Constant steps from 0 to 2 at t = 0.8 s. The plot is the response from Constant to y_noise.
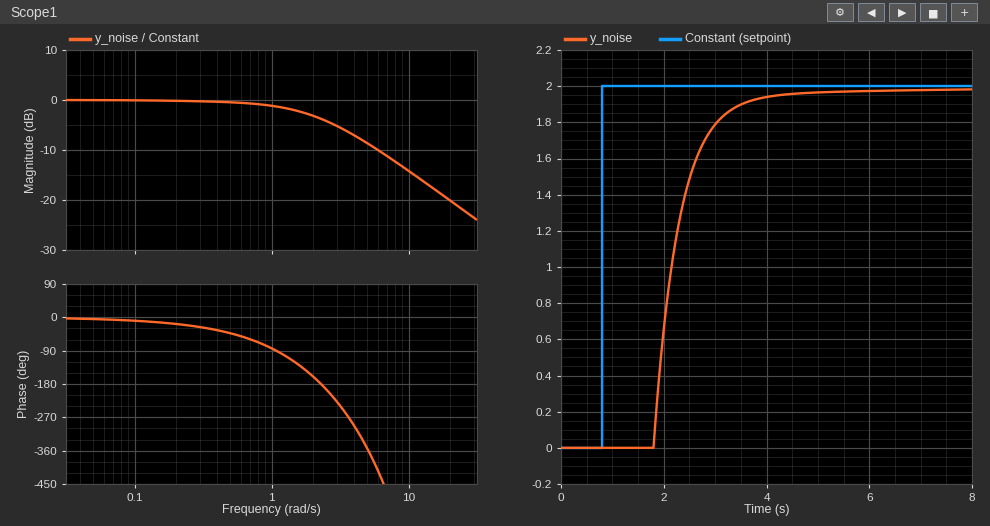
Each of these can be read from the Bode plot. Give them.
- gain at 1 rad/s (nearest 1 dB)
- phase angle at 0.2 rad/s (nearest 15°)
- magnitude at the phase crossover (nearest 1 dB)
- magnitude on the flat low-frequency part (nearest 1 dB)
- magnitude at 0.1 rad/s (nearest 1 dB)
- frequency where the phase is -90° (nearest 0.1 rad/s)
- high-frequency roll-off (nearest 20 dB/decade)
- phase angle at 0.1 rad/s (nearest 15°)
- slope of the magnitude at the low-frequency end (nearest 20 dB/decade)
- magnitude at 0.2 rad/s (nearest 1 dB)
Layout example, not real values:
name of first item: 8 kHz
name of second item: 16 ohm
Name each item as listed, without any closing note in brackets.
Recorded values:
gain at 1 rad/s: -1 dB
phase angle at 0.2 rad/s: -15°
magnitude at the phase crossover: -4 dB
magnitude on the flat low-frequency part: 0 dB
magnitude at 0.1 rad/s: 0 dB
frequency where the phase is -90°: 1.1 rad/s
high-frequency roll-off: -20 dB/decade
phase angle at 0.1 rad/s: -15°
slope of the magnitude at the low-frequency end: 0 dB/decade
magnitude at 0.2 rad/s: 0 dB
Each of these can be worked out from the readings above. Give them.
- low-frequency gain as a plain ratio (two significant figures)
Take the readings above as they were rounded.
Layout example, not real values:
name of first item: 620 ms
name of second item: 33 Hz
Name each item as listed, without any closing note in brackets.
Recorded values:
low-frequency gain as a plain ratio: 1.0
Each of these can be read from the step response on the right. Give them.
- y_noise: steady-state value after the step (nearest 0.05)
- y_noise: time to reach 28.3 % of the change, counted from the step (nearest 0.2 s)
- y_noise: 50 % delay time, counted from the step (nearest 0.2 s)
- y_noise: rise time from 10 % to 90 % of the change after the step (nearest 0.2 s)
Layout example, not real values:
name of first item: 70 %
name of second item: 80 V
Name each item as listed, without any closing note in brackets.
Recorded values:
y_noise: steady-state value after the step: 2.00
y_noise: time to reach 28.3 % of the change, counted from the step: 1.2 s
y_noise: 50 % delay time, counted from the step: 1.4 s
y_noise: rise time from 10 % to 90 % of the change after the step: 1.2 s
